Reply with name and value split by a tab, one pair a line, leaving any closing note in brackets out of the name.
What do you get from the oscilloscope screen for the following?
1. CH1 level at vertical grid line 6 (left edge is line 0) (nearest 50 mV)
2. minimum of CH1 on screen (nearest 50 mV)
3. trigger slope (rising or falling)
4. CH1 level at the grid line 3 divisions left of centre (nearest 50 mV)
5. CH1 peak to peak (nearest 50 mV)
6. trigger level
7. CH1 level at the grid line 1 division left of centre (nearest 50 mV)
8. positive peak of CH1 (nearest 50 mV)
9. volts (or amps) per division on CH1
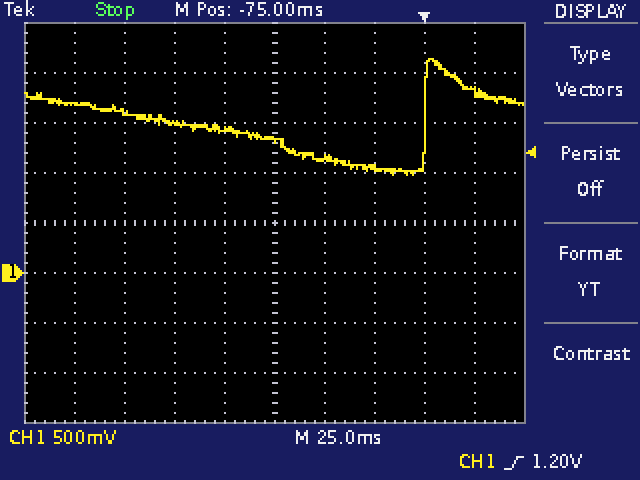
CH1 level at vertical grid line 6 (left edge is line 0)	1.15 V
minimum of CH1 on screen	1.00 V
trigger slope	rising
CH1 level at the grid line 3 divisions left of centre	1.60 V
CH1 peak to peak	1.15 V
trigger level	1.20 V
CH1 level at the grid line 1 division left of centre	1.45 V
positive peak of CH1	2.15 V
volts (or amps) per division on CH1	500 mV
